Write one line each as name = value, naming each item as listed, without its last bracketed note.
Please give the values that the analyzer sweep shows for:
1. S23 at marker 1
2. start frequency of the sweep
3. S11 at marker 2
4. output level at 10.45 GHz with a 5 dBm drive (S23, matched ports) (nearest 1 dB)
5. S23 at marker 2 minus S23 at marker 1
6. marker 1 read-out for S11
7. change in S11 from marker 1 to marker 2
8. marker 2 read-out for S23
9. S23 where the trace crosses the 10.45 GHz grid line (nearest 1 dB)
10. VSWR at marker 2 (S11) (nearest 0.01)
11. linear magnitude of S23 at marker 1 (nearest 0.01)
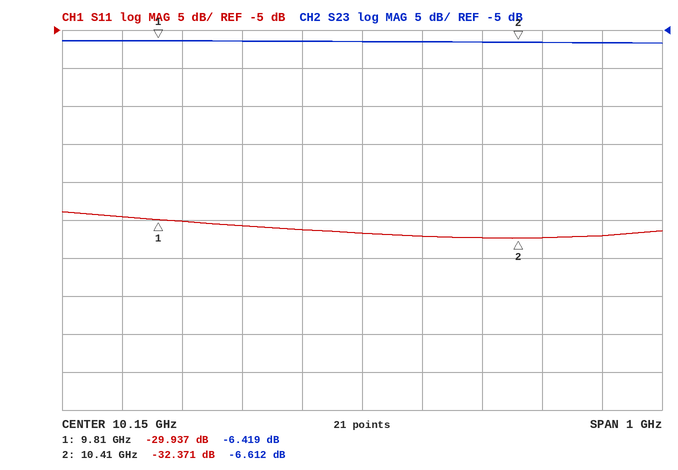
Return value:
S23 at marker 1 = -6.419 dB
start frequency of the sweep = 9.65 GHz
S11 at marker 2 = -32.371 dB
output level at 10.45 GHz with a 5 dBm drive (S23, matched ports) = -2 dBm
S23 at marker 2 minus S23 at marker 1 = -0.193 dB
marker 1 read-out for S11 = -29.937 dB
change in S11 from marker 1 to marker 2 = -2.434 dB
marker 2 read-out for S23 = -6.612 dB
S23 where the trace crosses the 10.45 GHz grid line = -7 dB
VSWR at marker 2 (S11) = 1.05
linear magnitude of S23 at marker 1 = 0.48
